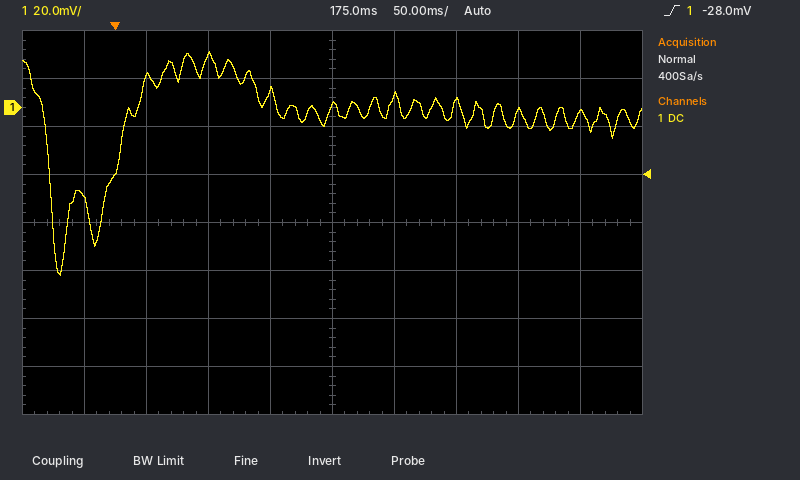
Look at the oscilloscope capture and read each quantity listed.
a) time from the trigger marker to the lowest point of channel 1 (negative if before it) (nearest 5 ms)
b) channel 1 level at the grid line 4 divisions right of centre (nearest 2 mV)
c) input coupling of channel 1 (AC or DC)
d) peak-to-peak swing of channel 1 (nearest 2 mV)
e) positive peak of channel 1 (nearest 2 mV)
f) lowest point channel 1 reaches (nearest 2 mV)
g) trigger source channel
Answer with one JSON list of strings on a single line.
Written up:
["-45 ms", "-2 mV", "DC", "94 mV", "24 mV", "-70 mV", "channel 1"]
